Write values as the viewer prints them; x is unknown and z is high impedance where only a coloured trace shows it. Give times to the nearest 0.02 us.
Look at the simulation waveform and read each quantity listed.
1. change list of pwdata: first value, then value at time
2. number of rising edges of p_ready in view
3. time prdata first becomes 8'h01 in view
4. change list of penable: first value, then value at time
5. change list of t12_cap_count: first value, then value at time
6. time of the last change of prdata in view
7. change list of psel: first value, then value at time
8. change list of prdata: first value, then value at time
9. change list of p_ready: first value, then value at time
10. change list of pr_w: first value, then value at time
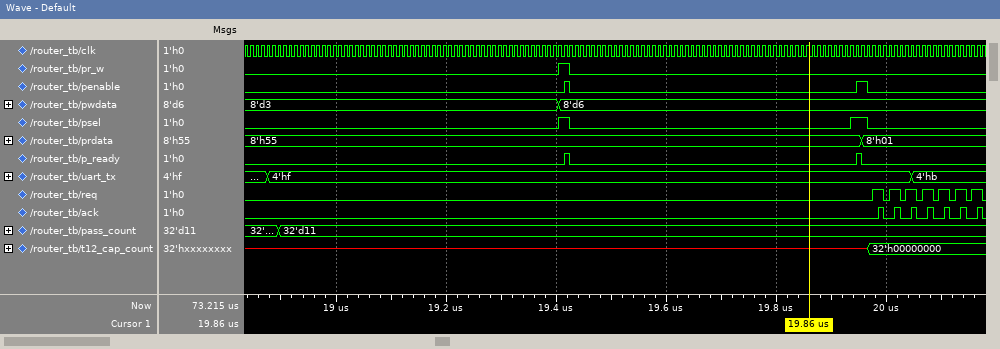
8'd3, 8'd6 at 19.4 us
2
19.96 us
0, 1 at 19.42 us, 0 at 19.42 us, 1 at 19.94 us, 0 at 19.96 us
x, 32'h00000000 at 19.96 us
19.96 us
0, 1 at 19.4 us, 0 at 19.42 us, 1 at 19.94 us, 0 at 19.96 us
8'h55, 8'h01 at 19.96 us
0, 1 at 19.42 us, 0 at 19.42 us, 1 at 19.94 us, 0 at 19.96 us
0, 1 at 19.4 us, 0 at 19.42 us
